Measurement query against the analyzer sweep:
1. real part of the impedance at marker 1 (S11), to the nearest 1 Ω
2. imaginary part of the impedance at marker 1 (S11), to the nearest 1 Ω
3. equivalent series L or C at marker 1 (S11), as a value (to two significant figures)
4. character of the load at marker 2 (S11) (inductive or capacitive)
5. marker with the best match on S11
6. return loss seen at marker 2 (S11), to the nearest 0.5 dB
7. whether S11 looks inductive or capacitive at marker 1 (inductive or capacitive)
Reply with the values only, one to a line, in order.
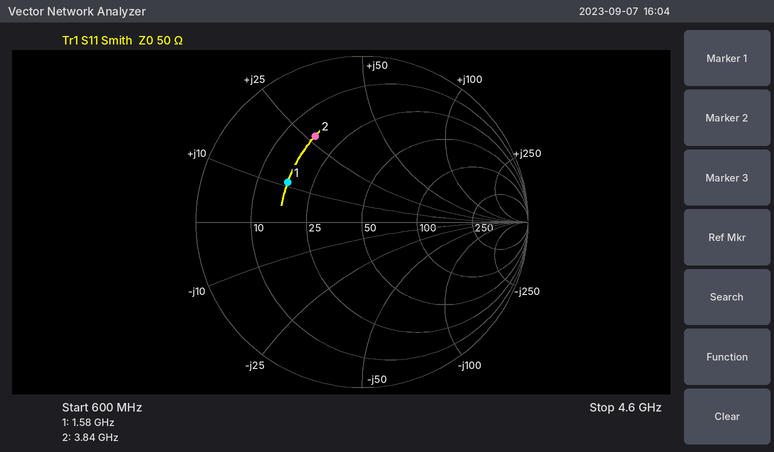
17 Ω
+11 Ω
1.1 nH
inductive
marker 1
4.5 dB
inductive
